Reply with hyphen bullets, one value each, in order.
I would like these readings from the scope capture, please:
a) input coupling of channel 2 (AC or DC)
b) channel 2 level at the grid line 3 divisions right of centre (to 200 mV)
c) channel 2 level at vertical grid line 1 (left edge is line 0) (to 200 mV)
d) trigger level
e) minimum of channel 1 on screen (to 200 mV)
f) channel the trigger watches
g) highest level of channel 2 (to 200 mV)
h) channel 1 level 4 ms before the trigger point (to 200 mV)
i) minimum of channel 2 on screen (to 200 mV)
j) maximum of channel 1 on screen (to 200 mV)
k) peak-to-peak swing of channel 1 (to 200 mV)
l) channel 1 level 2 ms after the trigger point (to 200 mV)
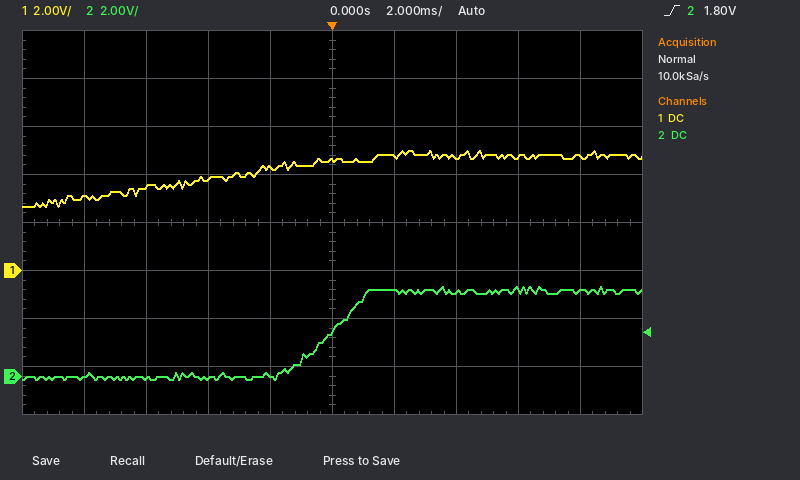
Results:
- DC
- 3.6 V
- 0.0 V
- 1.80 V
- 2.6 V
- channel 2
- 3.8 V
- 3.8 V
- -200 mV
- 5.0 V
- 2.4 V
- 4.8 V
